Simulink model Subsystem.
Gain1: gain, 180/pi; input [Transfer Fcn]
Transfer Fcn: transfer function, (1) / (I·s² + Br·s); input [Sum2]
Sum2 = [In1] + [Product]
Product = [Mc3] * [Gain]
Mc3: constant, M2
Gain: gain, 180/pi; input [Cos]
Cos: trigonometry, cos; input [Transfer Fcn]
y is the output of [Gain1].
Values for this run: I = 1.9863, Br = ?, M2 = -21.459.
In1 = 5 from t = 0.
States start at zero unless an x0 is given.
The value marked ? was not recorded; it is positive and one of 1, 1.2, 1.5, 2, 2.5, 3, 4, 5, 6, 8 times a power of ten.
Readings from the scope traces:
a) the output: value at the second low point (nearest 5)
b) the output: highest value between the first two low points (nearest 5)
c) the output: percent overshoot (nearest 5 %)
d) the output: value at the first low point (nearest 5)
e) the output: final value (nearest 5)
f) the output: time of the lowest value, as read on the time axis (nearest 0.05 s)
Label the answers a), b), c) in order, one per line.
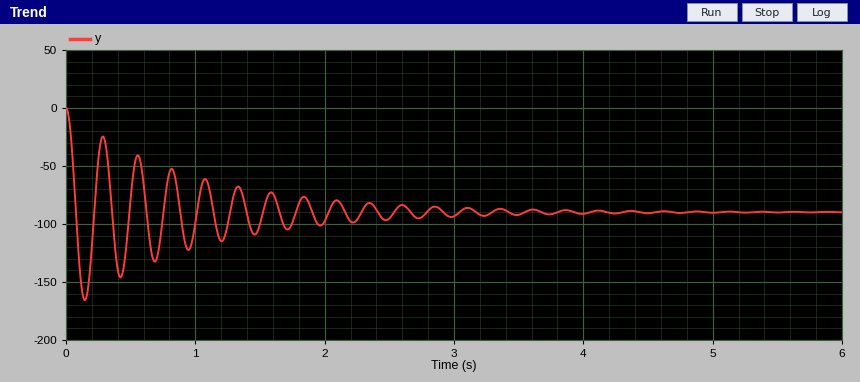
a) -145
b) -25
c) 85 %
d) -165
e) -90
f) 0.15 s
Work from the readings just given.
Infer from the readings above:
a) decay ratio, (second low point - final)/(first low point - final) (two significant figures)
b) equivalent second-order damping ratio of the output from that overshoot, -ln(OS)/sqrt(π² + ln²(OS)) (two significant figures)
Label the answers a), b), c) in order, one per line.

a) 0.73
b) 0.052
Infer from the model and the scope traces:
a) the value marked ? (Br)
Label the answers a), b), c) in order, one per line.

a) 4
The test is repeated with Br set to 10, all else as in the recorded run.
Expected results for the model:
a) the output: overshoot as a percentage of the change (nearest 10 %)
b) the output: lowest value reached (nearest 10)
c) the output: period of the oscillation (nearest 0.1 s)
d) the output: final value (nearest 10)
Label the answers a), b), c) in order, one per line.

a) 70 %
b) -150
c) 0.3 s
d) -90
